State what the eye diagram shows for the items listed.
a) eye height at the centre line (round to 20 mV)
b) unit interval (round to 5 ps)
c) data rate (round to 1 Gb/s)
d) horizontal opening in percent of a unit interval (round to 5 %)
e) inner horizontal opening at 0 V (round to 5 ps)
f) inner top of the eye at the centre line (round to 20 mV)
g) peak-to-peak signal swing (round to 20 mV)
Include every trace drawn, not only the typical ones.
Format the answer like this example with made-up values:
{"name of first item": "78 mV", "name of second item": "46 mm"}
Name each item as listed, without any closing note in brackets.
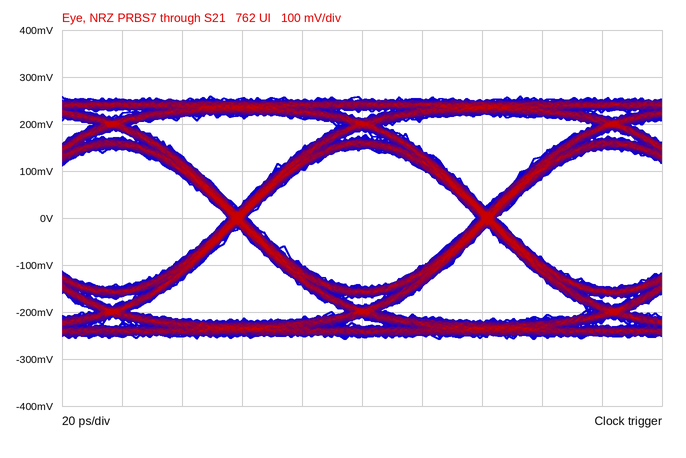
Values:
{"eye height at the centre line": "300 mV", "unit interval": "85 ps", "data rate": "12 Gb/s", "horizontal opening in percent of a unit interval": "90 %", "inner horizontal opening at 0 V": "75 ps", "inner top of the eye at the centre line": "140 mV", "peak-to-peak signal swing": "520 mV"}
